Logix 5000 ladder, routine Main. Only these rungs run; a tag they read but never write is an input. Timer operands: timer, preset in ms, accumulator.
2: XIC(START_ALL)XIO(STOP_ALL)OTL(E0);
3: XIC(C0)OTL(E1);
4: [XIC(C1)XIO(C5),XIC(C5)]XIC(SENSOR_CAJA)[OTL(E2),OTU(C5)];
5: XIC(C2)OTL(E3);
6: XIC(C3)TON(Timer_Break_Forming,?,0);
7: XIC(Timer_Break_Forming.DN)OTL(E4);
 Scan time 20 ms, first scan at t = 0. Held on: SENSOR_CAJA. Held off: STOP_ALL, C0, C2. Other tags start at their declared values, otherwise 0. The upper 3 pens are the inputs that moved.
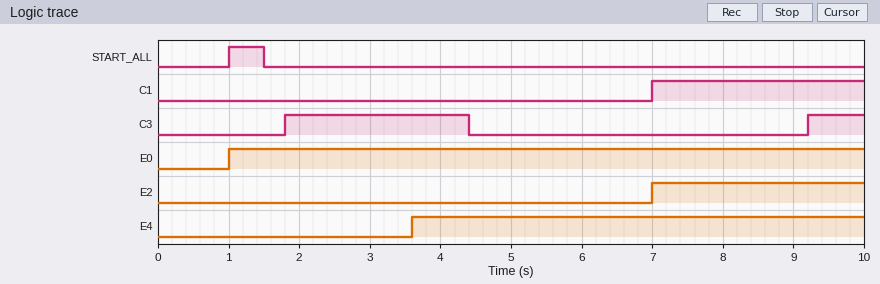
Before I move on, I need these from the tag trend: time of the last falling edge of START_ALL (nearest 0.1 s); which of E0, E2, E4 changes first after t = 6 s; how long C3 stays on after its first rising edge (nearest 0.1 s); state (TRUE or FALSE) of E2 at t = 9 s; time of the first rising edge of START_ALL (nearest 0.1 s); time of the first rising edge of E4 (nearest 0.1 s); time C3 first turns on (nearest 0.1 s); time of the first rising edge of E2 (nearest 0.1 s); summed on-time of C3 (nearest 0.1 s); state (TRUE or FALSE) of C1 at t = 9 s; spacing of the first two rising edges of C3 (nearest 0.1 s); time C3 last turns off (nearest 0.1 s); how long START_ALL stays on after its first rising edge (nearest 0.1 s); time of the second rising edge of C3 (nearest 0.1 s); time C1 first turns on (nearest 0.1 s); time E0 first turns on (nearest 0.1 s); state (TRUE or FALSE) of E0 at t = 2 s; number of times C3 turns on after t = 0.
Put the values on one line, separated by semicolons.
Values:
1.5 s; E2; 2.6 s; TRUE; 1.0 s; 3.6 s; 1.8 s; 7.0 s; 3.4 s; TRUE; 7.4 s; 4.4 s; 0.5 s; 9.2 s; 7.0 s; 1.0 s; TRUE; 2
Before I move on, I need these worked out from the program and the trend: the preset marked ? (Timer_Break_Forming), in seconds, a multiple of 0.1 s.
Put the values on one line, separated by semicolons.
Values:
1.8 s
